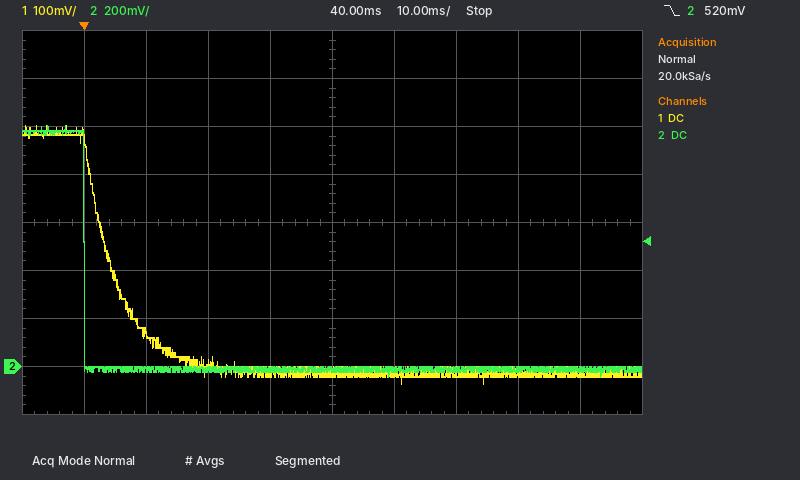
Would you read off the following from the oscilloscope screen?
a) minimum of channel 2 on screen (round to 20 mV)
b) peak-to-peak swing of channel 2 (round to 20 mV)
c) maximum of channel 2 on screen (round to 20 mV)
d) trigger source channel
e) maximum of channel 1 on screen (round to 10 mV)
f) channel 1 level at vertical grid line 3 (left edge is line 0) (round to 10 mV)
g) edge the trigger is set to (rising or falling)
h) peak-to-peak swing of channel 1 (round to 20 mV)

-40 mV
1.04 V
1.00 V
channel 2
500 mV
10 mV
falling
540 mV
